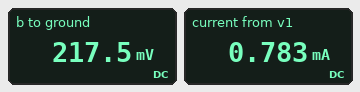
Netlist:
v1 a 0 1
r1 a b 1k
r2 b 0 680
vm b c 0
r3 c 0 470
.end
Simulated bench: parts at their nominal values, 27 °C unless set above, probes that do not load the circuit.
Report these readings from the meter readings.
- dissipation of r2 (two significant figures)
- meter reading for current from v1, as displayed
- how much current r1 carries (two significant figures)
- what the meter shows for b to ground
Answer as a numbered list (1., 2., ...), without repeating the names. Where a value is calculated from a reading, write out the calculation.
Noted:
1. (217.5 mV)^2 / 680 Ω = 70 µW
2. 0.783 mA
3. (1 V - 217.5 mV) / 1 kΩ = 780 µA
4. 217.5 mV
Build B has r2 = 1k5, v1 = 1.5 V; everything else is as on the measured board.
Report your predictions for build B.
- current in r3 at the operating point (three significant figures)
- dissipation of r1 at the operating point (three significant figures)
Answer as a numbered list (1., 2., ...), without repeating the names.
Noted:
1. 841 µA
2. 1.22 mW
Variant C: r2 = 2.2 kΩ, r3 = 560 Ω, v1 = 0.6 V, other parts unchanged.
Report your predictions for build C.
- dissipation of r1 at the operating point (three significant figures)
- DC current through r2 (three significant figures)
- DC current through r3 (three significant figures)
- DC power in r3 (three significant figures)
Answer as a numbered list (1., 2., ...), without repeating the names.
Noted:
1. 172 µW
2. 84.2 µA
3. 331 µA
4. 61.2 µW
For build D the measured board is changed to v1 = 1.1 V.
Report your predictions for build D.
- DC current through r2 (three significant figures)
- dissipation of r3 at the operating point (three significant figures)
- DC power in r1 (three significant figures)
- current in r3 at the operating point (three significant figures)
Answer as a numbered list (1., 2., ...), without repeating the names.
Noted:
1. 352 µA
2. 122 µW
3. 741 µW
4. 509 µA
